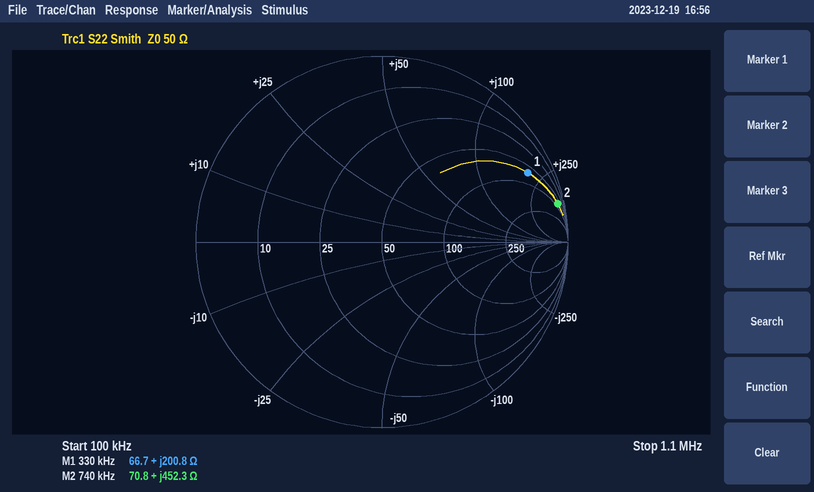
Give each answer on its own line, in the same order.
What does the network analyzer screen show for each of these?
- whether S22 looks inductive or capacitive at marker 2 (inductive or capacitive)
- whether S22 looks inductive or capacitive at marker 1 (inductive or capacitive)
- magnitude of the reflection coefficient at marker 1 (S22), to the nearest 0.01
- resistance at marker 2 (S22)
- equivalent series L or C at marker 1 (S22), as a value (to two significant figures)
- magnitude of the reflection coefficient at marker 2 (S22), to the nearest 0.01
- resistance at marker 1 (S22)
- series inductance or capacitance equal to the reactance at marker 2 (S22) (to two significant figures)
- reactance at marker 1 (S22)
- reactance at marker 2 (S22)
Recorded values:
inductive
inductive
0.87
70.8 Ω
97 µH
0.97
66.7 Ω
97 µH
+200.8 Ω
+452.3 Ω
